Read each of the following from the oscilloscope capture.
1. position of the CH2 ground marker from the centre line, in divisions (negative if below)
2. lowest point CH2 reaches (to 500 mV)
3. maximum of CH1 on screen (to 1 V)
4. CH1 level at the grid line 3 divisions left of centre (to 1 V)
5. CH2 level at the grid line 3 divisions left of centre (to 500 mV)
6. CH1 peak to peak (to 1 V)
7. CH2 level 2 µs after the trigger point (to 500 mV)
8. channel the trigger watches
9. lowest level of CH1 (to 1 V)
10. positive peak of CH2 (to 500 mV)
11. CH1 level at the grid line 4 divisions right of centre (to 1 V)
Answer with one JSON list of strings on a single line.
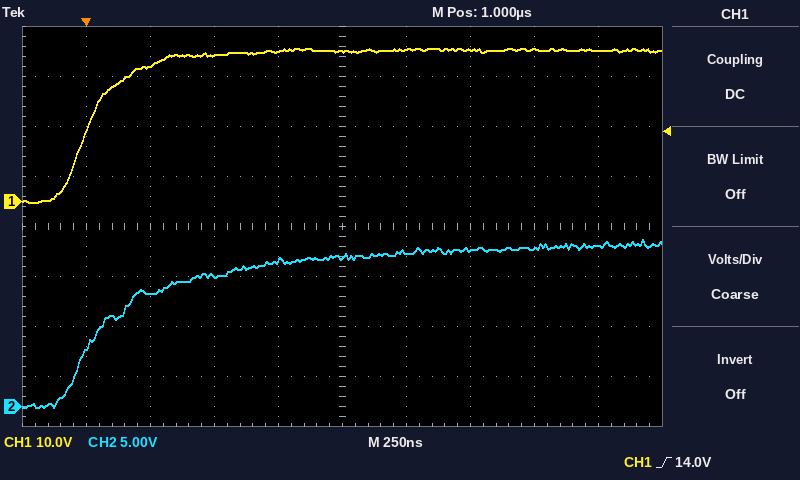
["-3.6 div", "0.0 V", "31 V", "27 V", "11.5 V", "31 V", "16.0 V", "CH1", "0 V", "16.5 V", "30 V"]
